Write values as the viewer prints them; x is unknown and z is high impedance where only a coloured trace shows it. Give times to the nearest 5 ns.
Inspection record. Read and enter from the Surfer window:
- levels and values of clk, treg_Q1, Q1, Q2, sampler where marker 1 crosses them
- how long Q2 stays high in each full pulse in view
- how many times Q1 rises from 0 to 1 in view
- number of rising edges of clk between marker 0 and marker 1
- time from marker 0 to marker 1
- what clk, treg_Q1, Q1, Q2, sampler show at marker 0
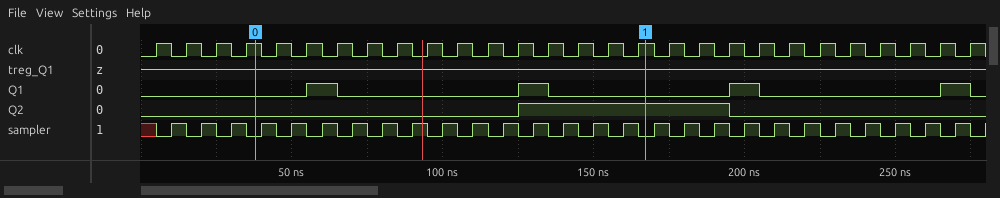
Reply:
clk=1, treg_Q1=z, Q1=0, Q2=1, sampler=0
70 ns
4
13
130 ns
clk=1, treg_Q1=z, Q1=0, Q2=0, sampler=0
